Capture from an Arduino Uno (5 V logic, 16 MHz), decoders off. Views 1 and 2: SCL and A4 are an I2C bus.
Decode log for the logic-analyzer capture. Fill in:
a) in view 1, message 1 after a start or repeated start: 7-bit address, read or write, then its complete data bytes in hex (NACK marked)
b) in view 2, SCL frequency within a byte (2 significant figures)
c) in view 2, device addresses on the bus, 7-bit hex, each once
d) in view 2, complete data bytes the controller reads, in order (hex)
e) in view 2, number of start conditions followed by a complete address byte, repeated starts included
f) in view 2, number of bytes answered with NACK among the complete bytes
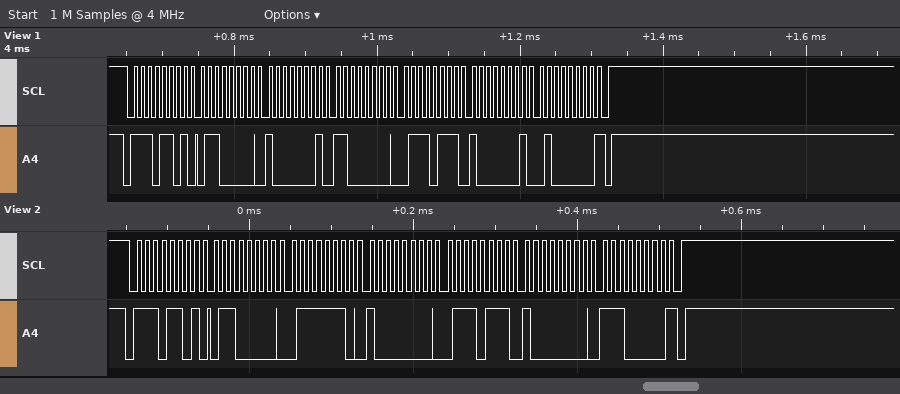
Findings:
0x76 read: 60 81 C0 77 81 40 NACK
100 kHz
0x76
60 7E 80 77 80 E0
1
1
